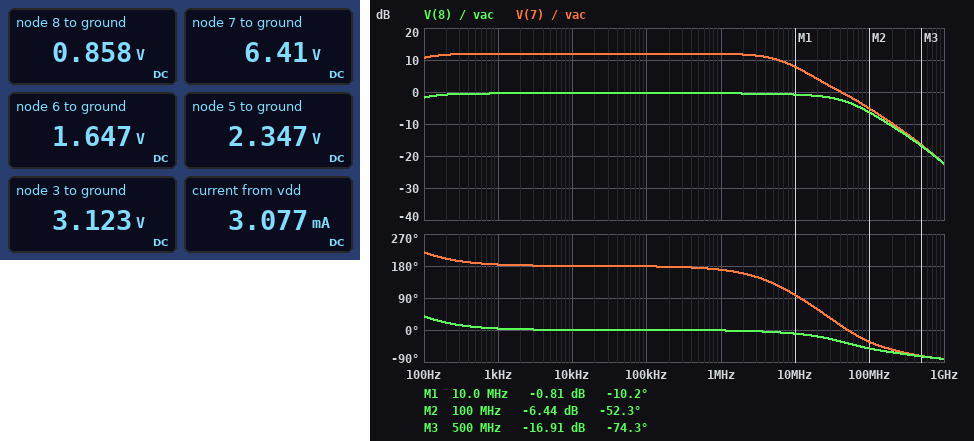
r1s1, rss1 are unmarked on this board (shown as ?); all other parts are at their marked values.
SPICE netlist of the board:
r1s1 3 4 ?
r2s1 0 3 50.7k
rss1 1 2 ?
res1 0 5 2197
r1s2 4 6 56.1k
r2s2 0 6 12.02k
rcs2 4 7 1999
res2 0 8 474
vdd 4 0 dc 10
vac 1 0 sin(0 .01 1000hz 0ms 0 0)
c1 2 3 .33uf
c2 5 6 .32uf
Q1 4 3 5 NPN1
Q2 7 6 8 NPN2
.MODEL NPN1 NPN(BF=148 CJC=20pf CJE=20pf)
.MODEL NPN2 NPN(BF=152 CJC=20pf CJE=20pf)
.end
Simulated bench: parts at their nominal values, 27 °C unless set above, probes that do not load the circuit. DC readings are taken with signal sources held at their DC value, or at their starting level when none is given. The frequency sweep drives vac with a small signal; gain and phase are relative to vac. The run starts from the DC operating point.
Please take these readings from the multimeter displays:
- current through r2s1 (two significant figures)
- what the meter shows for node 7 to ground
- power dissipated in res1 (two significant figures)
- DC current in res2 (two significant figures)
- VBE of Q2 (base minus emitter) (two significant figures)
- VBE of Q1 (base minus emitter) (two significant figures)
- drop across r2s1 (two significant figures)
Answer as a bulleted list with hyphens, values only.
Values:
- 62 µA
- 6.41 V
- 2.5 mW
- 1.8 mA
- 790 mV
- 780 mV
- 3.1 V
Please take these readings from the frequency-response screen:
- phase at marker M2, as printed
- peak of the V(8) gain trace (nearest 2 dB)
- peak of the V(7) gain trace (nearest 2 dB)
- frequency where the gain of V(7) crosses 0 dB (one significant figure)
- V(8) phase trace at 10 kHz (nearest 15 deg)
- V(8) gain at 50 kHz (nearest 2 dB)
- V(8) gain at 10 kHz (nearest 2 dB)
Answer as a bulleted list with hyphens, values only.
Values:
- -52.3 deg
- 0 dB
- 12 dB
- 40 MHz
- 0 deg
- 0 dB
- 0 dB
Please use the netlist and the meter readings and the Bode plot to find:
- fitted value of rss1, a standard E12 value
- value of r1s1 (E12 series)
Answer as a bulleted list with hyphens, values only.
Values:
- 220 Ω
- 100 kΩ
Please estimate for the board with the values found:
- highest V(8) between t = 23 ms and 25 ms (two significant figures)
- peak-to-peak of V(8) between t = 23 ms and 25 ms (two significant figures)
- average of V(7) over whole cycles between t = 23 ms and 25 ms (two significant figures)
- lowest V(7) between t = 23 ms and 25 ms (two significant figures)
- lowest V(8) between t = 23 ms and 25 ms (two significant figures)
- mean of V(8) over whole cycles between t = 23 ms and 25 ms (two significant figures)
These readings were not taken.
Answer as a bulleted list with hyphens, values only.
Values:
- 870 mV
- 19 mV
- 6.4 V
- 6.4 V
- 850 mV
- 860 mV
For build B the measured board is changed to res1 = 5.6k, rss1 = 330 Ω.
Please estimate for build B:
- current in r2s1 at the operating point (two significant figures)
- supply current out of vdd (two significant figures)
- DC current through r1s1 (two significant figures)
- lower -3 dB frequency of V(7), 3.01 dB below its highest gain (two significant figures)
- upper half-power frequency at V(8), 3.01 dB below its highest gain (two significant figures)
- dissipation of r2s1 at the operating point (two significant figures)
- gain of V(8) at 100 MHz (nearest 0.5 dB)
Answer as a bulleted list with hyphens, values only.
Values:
- 64 µA
- 2.5 mA
- 67 µA
- 60 Hz
- 26 MHz
- 210 µW
- -10.0 dB
